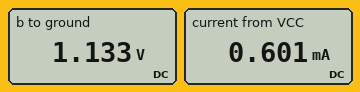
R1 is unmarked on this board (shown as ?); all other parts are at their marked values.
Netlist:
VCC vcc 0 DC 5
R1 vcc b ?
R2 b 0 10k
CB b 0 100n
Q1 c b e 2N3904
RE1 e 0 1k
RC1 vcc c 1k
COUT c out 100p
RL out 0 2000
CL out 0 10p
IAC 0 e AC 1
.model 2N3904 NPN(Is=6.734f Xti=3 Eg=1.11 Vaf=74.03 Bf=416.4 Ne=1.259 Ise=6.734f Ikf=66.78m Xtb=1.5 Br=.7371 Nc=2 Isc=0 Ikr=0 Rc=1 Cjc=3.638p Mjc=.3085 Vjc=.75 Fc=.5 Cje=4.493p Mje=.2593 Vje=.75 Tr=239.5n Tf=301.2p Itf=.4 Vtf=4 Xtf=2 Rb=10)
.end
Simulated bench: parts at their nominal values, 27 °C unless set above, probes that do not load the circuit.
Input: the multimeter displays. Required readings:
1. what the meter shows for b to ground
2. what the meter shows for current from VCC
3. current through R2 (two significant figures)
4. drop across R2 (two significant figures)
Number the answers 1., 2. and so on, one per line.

1. 1.133 V
2. 0.601 mA
3. 110 µA
4. 1.1 V
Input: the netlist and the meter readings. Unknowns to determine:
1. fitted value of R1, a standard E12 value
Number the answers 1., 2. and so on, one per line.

1. 33 kΩ
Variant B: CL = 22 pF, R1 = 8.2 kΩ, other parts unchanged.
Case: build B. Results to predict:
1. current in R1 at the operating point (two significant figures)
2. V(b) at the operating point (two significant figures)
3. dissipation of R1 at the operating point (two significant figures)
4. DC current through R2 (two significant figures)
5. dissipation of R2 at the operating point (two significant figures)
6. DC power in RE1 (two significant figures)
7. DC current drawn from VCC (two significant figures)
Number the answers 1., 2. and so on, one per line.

1. 280 µA
2. 2.7 V
3. 650 µW
4. 270 µA
5. 720 µW
6. 4.0 mW
7. 2.3 mA
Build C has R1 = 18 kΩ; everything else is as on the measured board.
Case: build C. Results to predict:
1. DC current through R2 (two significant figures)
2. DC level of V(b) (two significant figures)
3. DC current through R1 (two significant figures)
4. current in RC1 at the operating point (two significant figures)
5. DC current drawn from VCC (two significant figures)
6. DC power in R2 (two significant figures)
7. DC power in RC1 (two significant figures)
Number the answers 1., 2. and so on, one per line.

1. 170 µA
2. 1.7 V
3. 180 µA
4. 1.1 mA
5. 1.2 mA
6. 300 µW
7. 1.1 mW
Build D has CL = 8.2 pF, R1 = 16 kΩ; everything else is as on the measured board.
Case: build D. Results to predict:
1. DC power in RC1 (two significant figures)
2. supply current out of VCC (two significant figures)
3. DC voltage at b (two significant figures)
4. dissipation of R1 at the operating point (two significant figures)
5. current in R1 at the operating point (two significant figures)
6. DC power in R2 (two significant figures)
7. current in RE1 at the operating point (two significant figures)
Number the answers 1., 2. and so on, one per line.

1. 1.4 mW
2. 1.4 mA
3. 1.9 V
4. 610 µW
5. 200 µA
6. 350 µW
7. 1.2 mA
